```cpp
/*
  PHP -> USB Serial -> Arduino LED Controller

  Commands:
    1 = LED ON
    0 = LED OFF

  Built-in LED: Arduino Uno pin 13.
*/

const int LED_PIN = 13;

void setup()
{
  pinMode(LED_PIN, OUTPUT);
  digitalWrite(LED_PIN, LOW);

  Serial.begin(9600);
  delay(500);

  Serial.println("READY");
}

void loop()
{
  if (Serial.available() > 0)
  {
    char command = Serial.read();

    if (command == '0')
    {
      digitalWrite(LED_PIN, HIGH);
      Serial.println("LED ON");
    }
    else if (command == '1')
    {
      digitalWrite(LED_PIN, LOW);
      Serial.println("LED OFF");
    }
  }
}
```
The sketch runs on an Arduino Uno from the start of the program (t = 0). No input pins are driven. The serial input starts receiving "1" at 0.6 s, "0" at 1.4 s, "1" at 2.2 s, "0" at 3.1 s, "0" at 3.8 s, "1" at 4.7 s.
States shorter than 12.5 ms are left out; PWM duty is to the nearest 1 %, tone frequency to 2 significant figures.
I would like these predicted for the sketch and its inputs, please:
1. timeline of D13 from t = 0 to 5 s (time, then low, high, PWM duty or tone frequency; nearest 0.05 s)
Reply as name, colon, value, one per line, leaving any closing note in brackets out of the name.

timeline of D13 from t = 0 to 5 s: 0 s low; 1.4 s high; 2.2 s low; 3.1 s high; 4.7 s low
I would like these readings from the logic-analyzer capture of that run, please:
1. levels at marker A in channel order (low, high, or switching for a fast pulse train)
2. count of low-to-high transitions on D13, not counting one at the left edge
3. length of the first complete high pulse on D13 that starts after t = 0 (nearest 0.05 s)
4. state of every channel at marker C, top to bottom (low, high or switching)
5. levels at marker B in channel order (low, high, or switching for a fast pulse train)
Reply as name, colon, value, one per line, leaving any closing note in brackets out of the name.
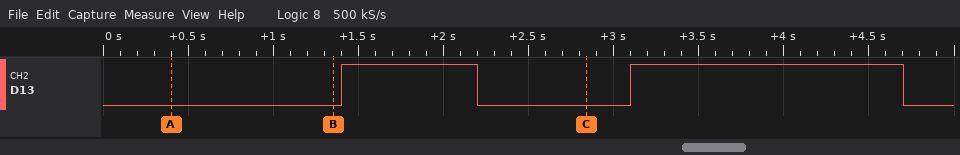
levels at marker A in channel order: D13 low
count of low-to-high transitions on D13, not counting one at the left edge: 2
length of the first complete high pulse on D13 that starts after t = 0: 0.80 s
state of every channel at marker C, top to bottom: D13 low
levels at marker B in channel order: D13 low
